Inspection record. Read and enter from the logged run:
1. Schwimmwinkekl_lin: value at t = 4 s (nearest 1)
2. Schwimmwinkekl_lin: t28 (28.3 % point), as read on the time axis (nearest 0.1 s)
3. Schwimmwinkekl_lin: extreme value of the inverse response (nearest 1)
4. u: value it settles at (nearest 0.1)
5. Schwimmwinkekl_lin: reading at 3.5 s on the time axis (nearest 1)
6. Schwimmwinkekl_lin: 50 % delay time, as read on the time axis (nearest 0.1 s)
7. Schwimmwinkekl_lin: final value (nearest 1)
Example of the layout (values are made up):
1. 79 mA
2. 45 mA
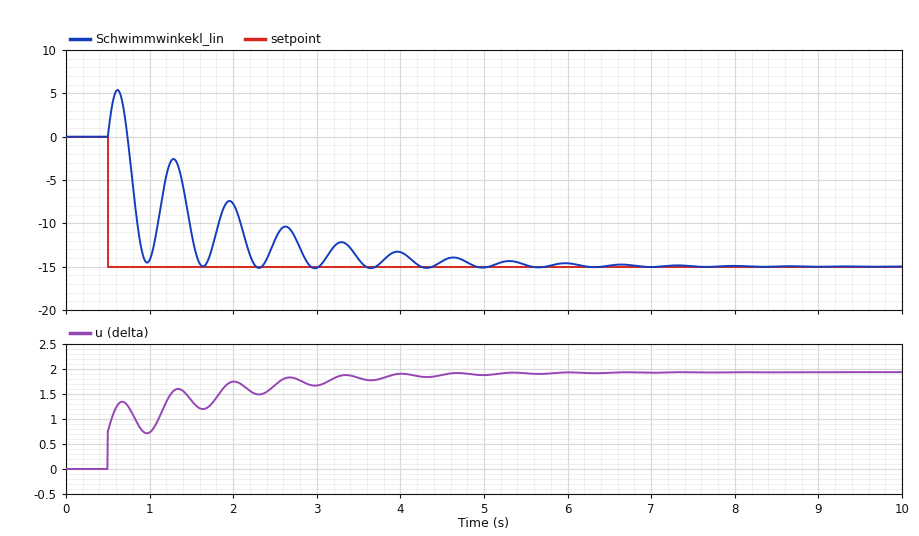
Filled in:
1. -13
2. 0.8 s
3. 5
4. 1.9
5. -14
6. 0.8 s
7. -15
